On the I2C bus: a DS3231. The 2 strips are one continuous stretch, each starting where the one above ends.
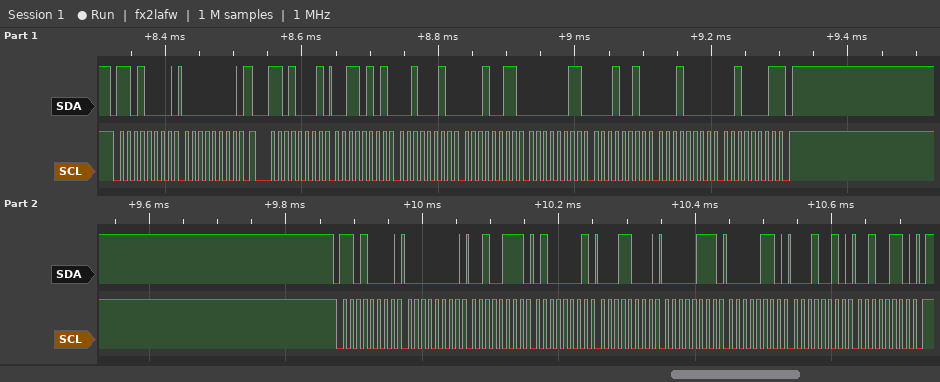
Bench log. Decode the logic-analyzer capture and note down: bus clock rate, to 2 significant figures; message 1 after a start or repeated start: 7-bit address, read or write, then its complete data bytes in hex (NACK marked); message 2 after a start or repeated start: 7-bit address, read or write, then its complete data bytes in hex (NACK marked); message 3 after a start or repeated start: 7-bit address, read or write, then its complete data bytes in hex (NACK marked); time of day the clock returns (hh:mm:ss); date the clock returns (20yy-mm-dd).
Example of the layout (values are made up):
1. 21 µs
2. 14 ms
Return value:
1. 100 kHz
2. 0x68 write: 00
3. 0x68 read: 35 22 13 03 12 10 21 NACK
4. 0x68 write: 00 27 41 18 07 06 12 26
5. 13:22:35
6. 2021-10-12
